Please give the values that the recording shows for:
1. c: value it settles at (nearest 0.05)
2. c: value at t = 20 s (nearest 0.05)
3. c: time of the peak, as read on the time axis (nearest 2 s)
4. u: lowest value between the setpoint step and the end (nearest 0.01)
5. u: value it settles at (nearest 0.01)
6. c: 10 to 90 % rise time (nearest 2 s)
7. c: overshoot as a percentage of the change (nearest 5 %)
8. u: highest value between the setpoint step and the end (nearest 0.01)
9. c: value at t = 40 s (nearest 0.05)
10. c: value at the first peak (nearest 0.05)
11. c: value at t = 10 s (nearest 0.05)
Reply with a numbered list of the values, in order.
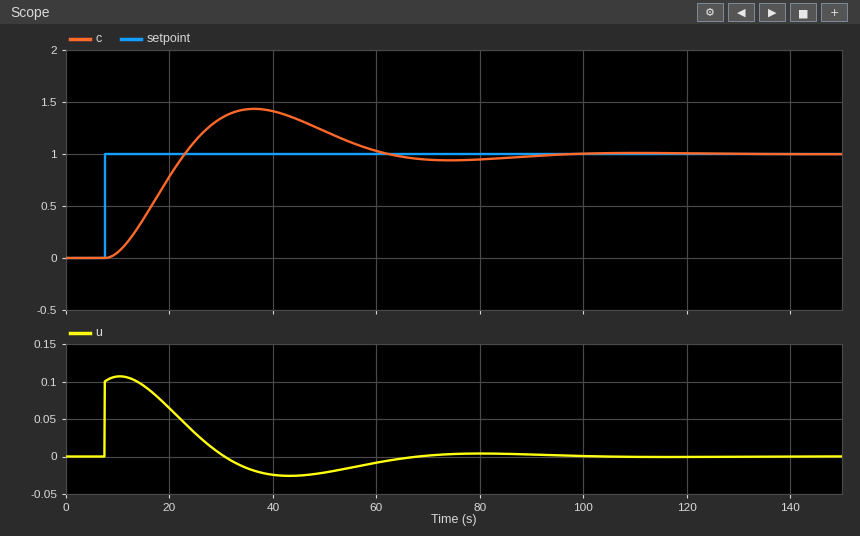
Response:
1. 1.00
2. 0.80
3. 36 s
4. -0.03
5. 0.00
6. 10 s
7. 45 %
8. 0.11
9. 1.40
10. 1.45
11. 0.05
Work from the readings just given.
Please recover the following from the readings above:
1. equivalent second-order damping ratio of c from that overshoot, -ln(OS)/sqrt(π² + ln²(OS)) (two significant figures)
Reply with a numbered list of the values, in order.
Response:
1. 0.25
